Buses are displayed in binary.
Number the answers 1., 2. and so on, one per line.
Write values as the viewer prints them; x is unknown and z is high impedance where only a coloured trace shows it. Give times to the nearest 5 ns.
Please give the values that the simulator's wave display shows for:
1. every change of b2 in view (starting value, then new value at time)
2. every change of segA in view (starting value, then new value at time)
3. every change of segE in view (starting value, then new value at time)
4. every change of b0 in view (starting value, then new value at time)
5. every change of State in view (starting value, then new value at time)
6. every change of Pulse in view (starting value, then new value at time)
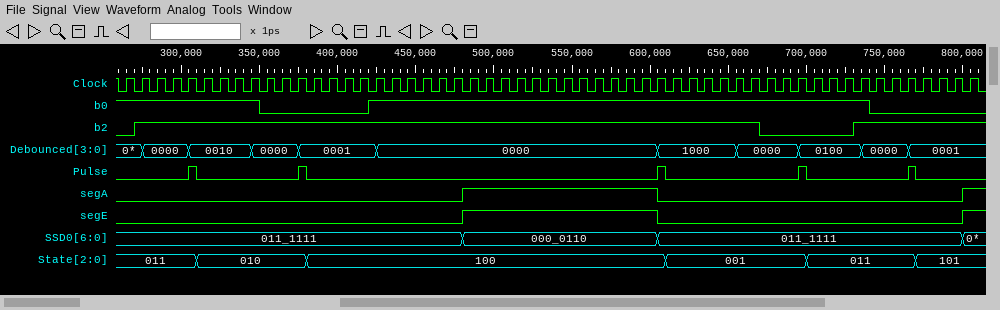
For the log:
1. 0, 1 at 270 ns, 0 at 670 ns, 1 at 730 ns
2. 0, 1 at 480 ns, 0 at 605 ns, 1 at 800 ns
3. 0, 1 at 480 ns, 0 at 605 ns, 1 at 800 ns
4. 1, 0 at 350 ns, 1 at 420 ns, 0 at 740 ns
5. 011, 010 at 310 ns, 100 at 380 ns, 001 at 610 ns, 011 at 700 ns, 101 at 770 ns
6. 0, 1 at 305 ns, 0 at 310 ns, 1 at 375 ns, 0 at 380 ns, 1 at 605 ns, 0 at 610 ns, 1 at 695 ns, 0 at 700 ns, 1 at 765 ns, 0 at 770 ns
